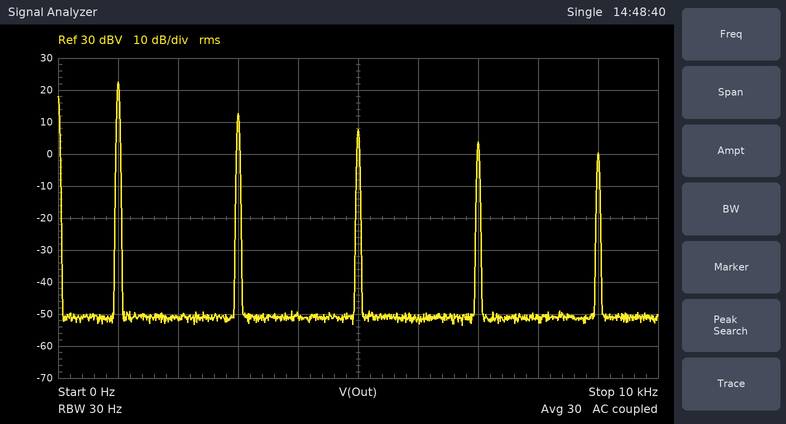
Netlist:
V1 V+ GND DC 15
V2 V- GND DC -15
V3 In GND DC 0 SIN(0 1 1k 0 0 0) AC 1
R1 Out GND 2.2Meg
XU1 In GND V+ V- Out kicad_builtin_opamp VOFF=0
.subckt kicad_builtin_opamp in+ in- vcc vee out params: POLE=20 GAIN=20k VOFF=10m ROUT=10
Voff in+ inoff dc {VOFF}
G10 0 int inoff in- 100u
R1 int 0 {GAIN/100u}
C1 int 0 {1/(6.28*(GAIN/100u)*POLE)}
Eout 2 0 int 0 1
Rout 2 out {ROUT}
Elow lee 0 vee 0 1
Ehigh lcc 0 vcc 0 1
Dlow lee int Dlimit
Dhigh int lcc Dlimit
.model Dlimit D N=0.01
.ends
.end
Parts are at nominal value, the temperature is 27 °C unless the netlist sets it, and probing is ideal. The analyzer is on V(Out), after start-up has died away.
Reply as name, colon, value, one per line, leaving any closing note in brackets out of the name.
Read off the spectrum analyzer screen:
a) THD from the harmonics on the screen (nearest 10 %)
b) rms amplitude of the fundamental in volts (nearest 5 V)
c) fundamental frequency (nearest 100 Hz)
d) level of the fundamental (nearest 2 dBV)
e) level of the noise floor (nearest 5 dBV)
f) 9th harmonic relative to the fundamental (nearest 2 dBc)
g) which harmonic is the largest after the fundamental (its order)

THD from the harmonics on the screen: 40 %
rms amplitude of the fundamental in volts: 15 V
fundamental frequency: 1.0 kHz
level of the fundamental: 22 dBV
level of the noise floor: -50 dBV
9th harmonic relative to the fundamental: -22 dBc
which harmonic is the largest after the fundamental: 3
